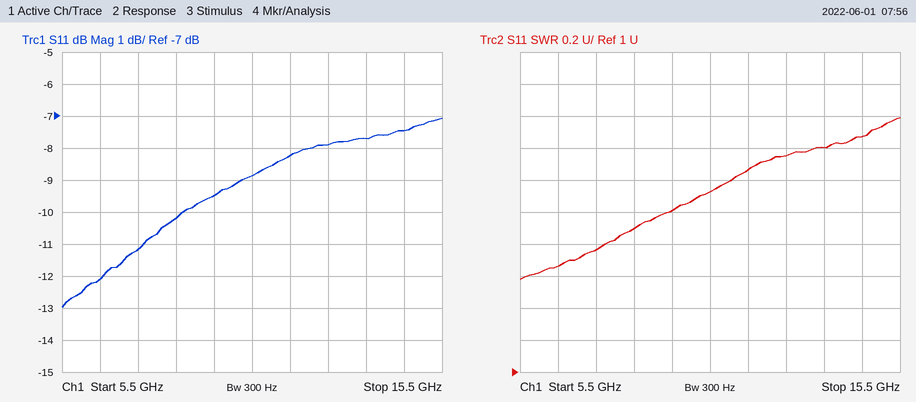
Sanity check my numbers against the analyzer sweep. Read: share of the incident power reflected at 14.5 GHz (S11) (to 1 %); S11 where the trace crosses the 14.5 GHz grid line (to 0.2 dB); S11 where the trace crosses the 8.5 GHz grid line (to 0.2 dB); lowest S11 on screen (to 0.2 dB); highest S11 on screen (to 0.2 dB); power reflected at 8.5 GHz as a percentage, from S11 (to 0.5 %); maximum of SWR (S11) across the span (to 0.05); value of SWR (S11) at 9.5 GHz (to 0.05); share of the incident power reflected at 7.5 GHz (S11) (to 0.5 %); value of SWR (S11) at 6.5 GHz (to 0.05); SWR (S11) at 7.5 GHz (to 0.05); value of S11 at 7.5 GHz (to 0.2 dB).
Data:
18 %
-7.4 dB
-10.2 dB
-13.0 dB
-7.0 dB
9.5 %
2.60
2.00
7.5 %
1.65
1.75
-11.2 dB
